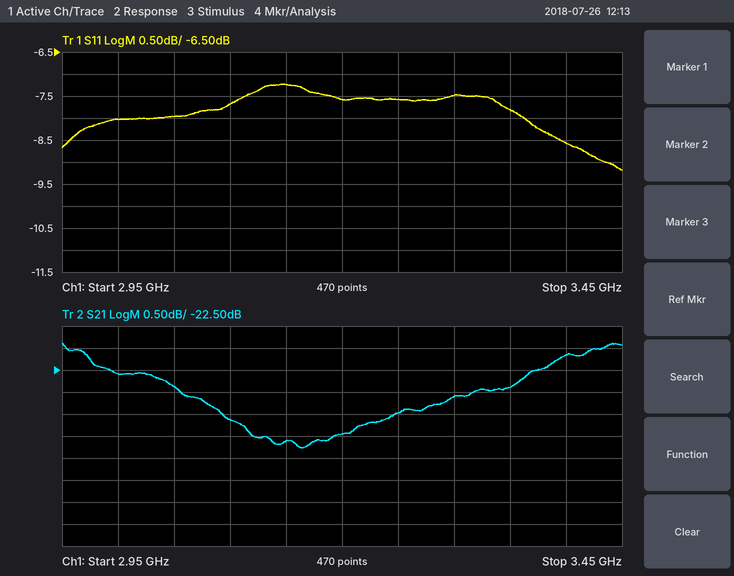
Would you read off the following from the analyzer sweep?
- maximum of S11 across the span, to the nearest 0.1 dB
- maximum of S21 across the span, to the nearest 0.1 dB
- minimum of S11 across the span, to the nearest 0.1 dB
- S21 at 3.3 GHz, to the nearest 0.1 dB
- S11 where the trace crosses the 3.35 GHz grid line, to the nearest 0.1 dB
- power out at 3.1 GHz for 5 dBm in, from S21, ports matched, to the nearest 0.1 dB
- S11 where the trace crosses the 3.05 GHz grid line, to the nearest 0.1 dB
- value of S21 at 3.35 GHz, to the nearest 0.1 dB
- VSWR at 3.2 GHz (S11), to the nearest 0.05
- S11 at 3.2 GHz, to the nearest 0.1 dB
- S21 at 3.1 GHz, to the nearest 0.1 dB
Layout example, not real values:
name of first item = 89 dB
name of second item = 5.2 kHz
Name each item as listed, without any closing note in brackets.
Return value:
maximum of S11 across the span, to the nearest 0.1 dB = -7.2 dB
maximum of S21 across the span, to the nearest 0.1 dB = -21.9 dB
minimum of S11 across the span, to the nearest 0.1 dB = -9.2 dB
S21 at 3.3 GHz, to the nearest 0.1 dB = -23.1 dB
S11 where the trace crosses the 3.35 GHz grid line, to the nearest 0.1 dB = -7.8 dB
power out at 3.1 GHz for 5 dBm in, from S21, ports matched, to the nearest 0.1 dB = -18.6 dBm
S11 where the trace crosses the 3.05 GHz grid line, to the nearest 0.1 dB = -8.0 dB
value of S21 at 3.35 GHz, to the nearest 0.1 dB = -22.9 dB
VSWR at 3.2 GHz (S11), to the nearest 0.05 = 2.45
S11 at 3.2 GHz, to the nearest 0.1 dB = -7.6 dB
S21 at 3.1 GHz, to the nearest 0.1 dB = -23.6 dB
